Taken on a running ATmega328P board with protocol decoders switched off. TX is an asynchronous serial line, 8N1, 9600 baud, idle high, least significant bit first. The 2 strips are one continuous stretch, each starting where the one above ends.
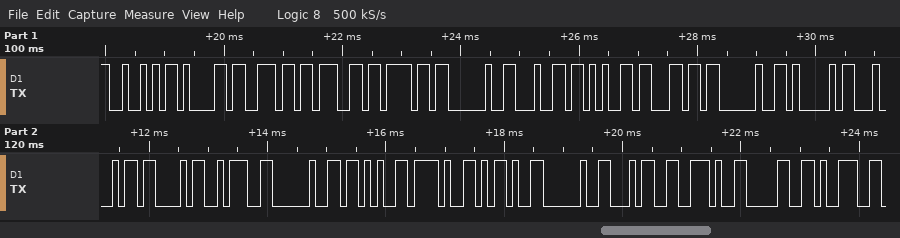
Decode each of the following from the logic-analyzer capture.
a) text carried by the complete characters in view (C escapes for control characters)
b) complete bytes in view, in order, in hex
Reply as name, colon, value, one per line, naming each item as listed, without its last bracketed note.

text carried by the complete characters in view: "Rango del ADC: +/- 4.09"
complete bytes in view, in order, in hex: 52 61 6E 67 6F 20 64 65 6C 20 41 44 43 3A 20 2B 2F 2D 20 34 2E 30 39
